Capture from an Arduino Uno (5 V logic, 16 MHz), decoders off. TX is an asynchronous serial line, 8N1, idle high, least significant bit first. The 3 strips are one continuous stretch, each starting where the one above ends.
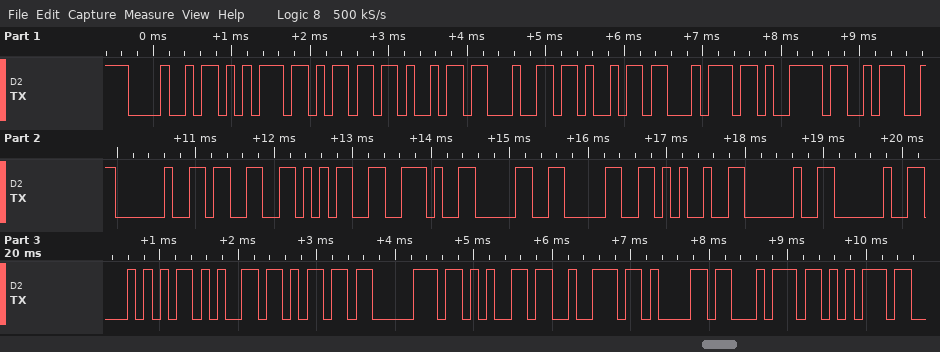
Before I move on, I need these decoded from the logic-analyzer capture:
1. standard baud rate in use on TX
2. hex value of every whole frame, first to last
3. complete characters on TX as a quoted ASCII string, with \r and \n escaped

9600 baud
48 75 6D 69 64 69 74 79 3A 20 33 35 2E 30 30 25 20 20 54 65 6D 70 65 72 61 74 75
"Humidity: 35.00%  Temperatu"
